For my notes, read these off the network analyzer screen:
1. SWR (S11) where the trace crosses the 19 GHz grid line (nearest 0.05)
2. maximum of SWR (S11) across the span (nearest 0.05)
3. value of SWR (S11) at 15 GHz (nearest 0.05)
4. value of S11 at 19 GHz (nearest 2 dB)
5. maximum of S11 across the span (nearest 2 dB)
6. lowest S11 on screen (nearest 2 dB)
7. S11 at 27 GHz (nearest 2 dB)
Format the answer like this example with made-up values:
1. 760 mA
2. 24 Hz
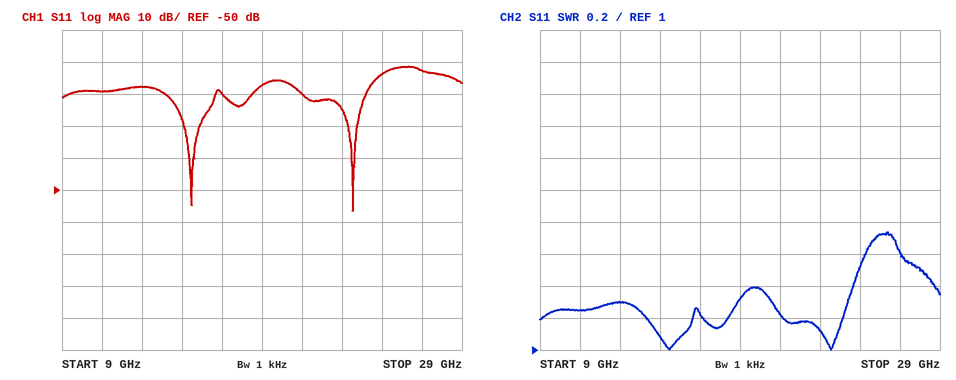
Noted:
1. 1.30
2. 1.75
3. 1.10
4. -18 dB
5. -12 dB
6. -56 dB
7. -12 dB
